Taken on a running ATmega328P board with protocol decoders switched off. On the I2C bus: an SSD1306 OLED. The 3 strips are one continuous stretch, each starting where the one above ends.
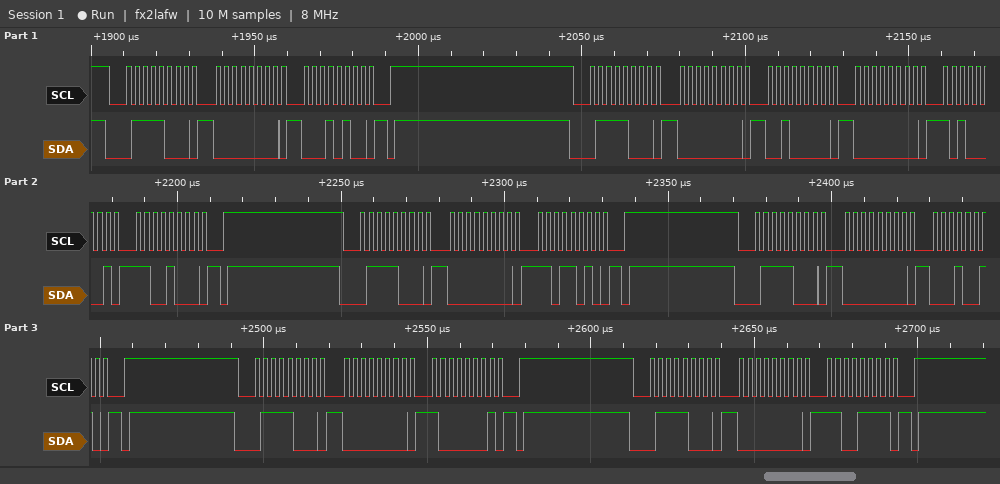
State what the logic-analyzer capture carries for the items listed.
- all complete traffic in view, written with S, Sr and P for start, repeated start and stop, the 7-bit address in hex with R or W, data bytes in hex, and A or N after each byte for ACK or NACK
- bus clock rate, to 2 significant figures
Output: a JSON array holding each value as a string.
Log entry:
["S 3CW A 00 A 14 A P S 3CW A 00 A 20 A 00 A A1 A C8 A P S 3CW A 00 A DA A P S 3CW A 00 A 12 A P S 3CW A 00 A 81 A P S 3CW A 00 A CF A P", "400 kHz"]
